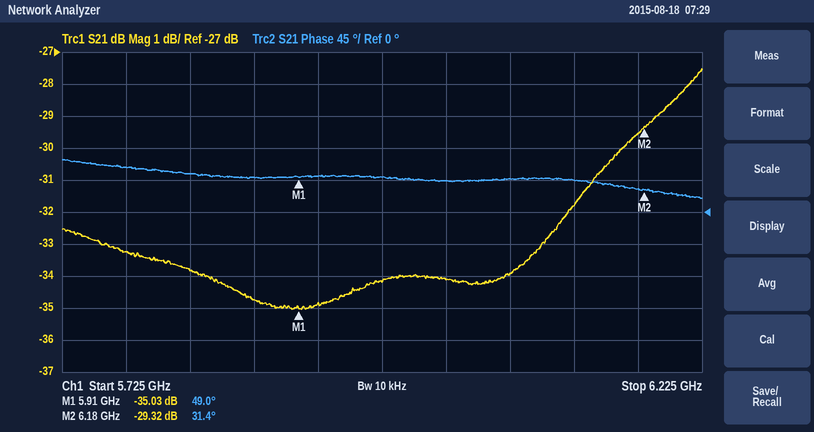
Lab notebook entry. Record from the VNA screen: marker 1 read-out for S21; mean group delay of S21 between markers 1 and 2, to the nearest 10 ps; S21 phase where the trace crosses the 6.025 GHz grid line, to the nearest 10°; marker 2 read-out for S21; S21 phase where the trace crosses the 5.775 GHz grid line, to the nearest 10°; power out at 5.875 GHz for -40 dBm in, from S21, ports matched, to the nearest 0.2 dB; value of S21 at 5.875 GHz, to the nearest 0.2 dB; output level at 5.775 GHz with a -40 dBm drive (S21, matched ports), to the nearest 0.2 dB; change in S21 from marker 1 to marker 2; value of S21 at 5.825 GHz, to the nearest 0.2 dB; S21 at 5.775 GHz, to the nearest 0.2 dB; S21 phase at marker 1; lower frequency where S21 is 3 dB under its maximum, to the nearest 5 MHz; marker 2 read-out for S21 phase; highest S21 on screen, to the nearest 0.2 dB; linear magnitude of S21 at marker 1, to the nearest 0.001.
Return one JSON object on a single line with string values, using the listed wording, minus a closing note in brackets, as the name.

{"marker 1 read-out for S21": "-35.03 dB", "mean group delay of S21 between markers 1 and 2, to the nearest 10 ps": "180 ps", "S21 phase where the trace crosses the 6.025 GHz grid line, to the nearest 10°": "40°", "marker 2 read-out for S21": "-29.32 dB", "S21 phase where the trace crosses the 5.775 GHz grid line, to the nearest 10°": "60°", "power out at 5.875 GHz for -40 dBm in, from S21, ports matched, to the nearest 0.2 dB": "-74.8 dBm", "value of S21 at 5.875 GHz, to the nearest 0.2 dB": "-34.8 dB", "output level at 5.775 GHz with a -40 dBm drive (S21, matched ports), to the nearest 0.2 dB": "-73.2 dBm", "change in S21 from marker 1 to marker 2": "5.71 dB", "value of S21 at 5.825 GHz, to the nearest 0.2 dB": "-33.8 dB", "S21 at 5.775 GHz, to the nearest 0.2 dB": "-33.2 dB", "S21 phase at marker 1": "49.0°", "lower frequency where S21 is 3 dB under its maximum, to the nearest 5 MHz": "6.150 GHz", "marker 2 read-out for S21 phase": "31.4°", "highest S21 on screen, to the nearest 0.2 dB": "-27.6 dB", "linear magnitude of S21 at marker 1, to the nearest 0.001": "0.018"}
